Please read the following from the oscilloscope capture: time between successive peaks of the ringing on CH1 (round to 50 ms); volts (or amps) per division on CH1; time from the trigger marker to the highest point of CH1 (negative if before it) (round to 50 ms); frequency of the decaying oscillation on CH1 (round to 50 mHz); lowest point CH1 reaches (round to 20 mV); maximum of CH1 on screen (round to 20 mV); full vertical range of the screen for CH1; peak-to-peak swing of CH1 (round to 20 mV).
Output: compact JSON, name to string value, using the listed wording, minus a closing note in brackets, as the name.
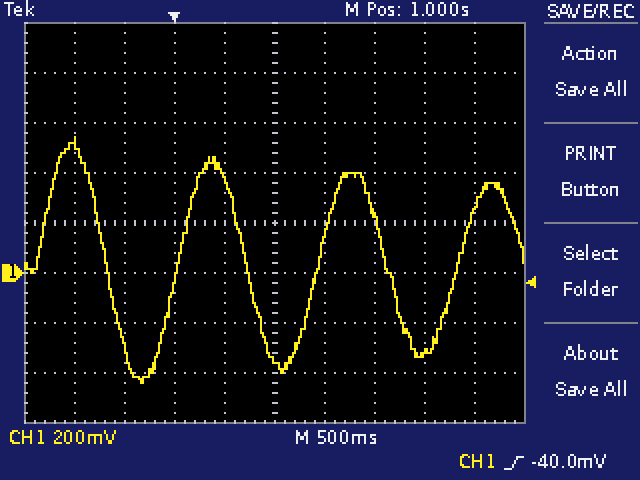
{"time between successive peaks of the ringing on CH1": "1.40 s", "volts (or amps) per division on CH1": "200 mV", "time from the trigger marker to the highest point of CH1 (negative if before it)": "-1.00 s", "frequency of the decaying oscillation on CH1": "700 mHz", "lowest point CH1 reaches": "-440 mV", "maximum of CH1 on screen": "540 mV", "full vertical range of the screen for CH1": "1.6 V", "peak-to-peak swing of CH1": "980 mV"}
